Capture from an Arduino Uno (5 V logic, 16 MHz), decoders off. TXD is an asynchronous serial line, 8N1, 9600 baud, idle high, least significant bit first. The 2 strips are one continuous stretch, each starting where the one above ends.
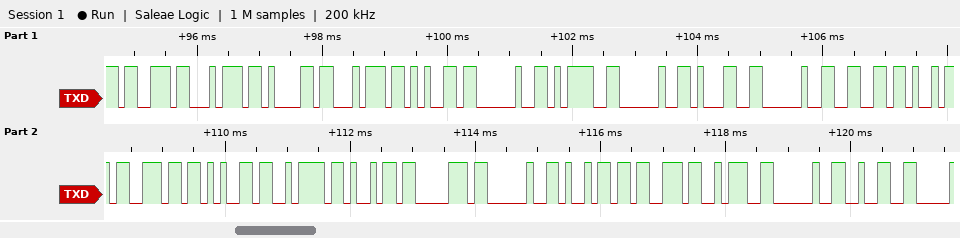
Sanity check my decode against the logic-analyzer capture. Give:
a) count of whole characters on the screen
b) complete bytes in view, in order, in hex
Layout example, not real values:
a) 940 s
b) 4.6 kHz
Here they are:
a) 23
b) 73 74 61 74 65 20 3D 20 31 20 66 69 6E 65 7A 69 70 20 69 73 3A 20 32
